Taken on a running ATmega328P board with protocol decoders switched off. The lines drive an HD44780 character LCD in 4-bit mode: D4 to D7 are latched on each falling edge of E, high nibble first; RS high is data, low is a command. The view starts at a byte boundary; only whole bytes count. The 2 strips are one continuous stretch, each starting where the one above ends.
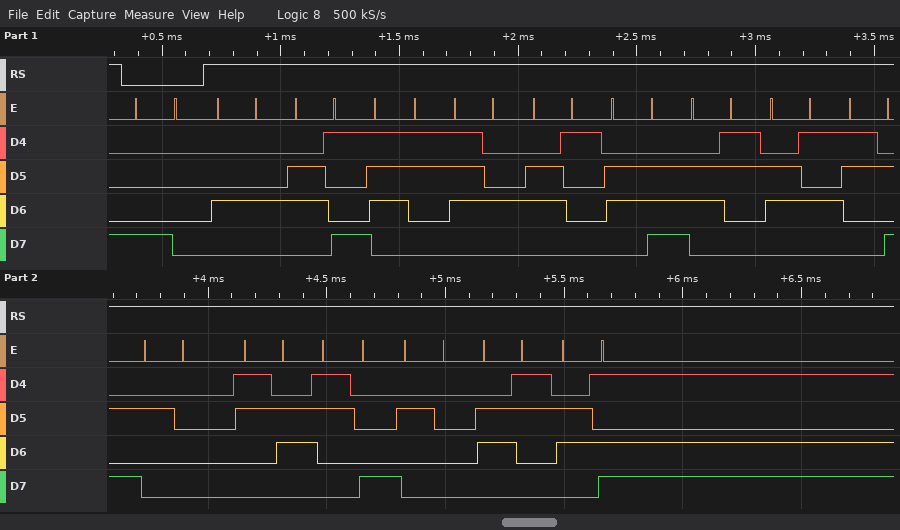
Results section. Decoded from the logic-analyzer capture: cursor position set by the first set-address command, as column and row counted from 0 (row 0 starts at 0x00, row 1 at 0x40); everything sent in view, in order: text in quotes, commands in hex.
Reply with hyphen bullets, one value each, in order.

- column 0, row 0
- 0x80 "Distance: 68 cm"
